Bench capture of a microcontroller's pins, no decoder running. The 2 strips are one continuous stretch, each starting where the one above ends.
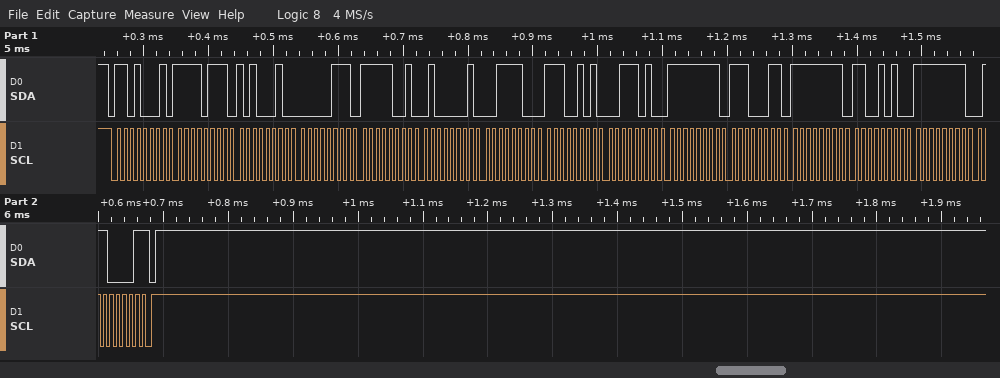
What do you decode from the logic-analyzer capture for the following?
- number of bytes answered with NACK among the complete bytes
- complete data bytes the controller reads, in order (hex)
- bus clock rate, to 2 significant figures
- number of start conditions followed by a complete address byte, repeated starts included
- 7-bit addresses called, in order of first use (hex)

1
F7 A2 07 F9 41 3C E5 3A FF E3 FF CA FF 61
100 kHz
1
0x68
